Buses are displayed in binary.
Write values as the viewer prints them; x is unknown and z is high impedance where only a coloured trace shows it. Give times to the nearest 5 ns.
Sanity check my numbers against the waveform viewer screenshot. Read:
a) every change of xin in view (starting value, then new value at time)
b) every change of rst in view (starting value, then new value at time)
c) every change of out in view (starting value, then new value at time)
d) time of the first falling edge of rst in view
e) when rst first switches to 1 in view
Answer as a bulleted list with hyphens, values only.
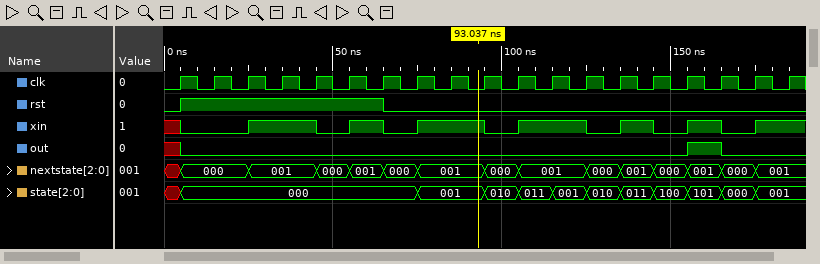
- x, 0 at 5 ns, 1 at 25 ns, 0 at 45 ns, 1 at 55 ns, 0 at 65 ns, 1 at 75 ns, 0 at 95 ns, 1 at 105 ns, 0 at 125 ns, 1 at 135 ns, 0 at 145 ns, 1 at 155 ns, 0 at 165 ns, 1 at 175 ns
- 0, 1 at 5 ns, 0 at 65 ns
- x, 0 at 5 ns, 1 at 155 ns, 0 at 165 ns
- 65 ns
- 5 ns
